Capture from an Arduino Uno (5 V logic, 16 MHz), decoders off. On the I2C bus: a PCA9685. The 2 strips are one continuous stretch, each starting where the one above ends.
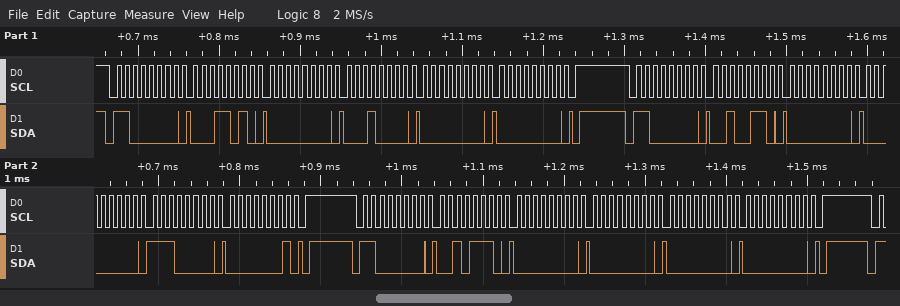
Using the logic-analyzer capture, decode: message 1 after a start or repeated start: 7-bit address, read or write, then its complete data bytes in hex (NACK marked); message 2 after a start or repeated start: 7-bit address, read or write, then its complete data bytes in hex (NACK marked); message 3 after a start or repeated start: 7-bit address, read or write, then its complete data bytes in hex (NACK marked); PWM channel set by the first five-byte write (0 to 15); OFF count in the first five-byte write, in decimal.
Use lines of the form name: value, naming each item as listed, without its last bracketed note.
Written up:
message 1 after a start or repeated start: 7-bit address, read or write, then its complete data bytes in hex: 0x60 write: 1A 00 10 00 00
message 2 after a start or repeated start: 7-bit address, read or write, then its complete data bytes in hex: 0x60 write: 26 00 00 E0 01
message 3 after a start or repeated start: 7-bit address, read or write, then its complete data bytes in hex: 0x60 write: 2E 00 00 00 00
PWM channel set by the first five-byte write: 5
OFF count in the first five-byte write, in decimal: 0
